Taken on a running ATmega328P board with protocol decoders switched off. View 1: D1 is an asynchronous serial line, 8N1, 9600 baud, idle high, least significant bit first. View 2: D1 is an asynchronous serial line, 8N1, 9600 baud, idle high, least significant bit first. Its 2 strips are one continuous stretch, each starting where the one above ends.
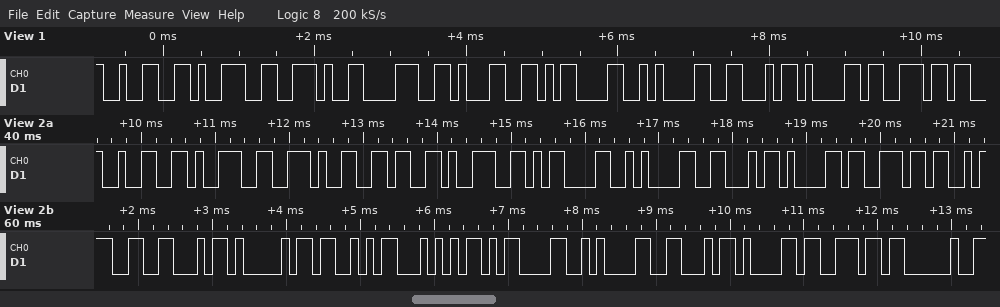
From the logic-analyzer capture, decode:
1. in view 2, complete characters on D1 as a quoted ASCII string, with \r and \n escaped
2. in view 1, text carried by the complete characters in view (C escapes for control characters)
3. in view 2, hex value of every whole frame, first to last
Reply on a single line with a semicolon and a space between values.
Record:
"29.69\r\nFan:FAST\r\nFan "; "29.81\r\nFan"; 32 39 2E 36 39 0D 0A 46 61 6E 3A 46 41 53 54 0D 0A 46 61 6E 20
